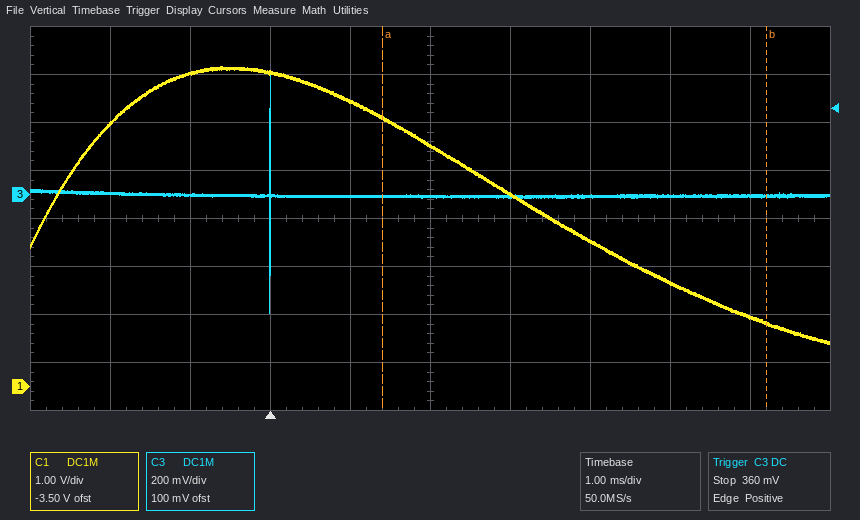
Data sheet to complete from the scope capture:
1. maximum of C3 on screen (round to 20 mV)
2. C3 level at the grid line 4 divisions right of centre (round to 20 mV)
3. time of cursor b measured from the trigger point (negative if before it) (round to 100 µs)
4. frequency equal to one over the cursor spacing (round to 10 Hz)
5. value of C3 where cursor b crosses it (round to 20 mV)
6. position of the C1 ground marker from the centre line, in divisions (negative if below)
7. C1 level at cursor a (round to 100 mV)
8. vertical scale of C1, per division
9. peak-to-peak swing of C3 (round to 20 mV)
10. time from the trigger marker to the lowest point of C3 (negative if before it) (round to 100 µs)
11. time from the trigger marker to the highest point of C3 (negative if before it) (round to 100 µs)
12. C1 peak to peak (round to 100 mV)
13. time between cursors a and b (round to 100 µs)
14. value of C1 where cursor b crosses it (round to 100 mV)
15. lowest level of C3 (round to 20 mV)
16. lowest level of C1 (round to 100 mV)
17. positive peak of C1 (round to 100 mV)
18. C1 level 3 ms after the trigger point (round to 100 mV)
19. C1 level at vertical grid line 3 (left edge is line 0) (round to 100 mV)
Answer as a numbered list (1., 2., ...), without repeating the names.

1. 500 mV
2. 0 mV
3. +6.2 ms
4. 210 Hz
5. 0 mV
6. -3.5 div
7. 5.6 V
8. 1 V
9. 1.00 V
10. 0.0 ms
11. 0.0 ms
12. 5.8 V
13. 4.8 ms
14. 1.3 V
15. -500 mV
16. 900 mV
17. 6.7 V
18. 4.0 V
19. 6.5 V
